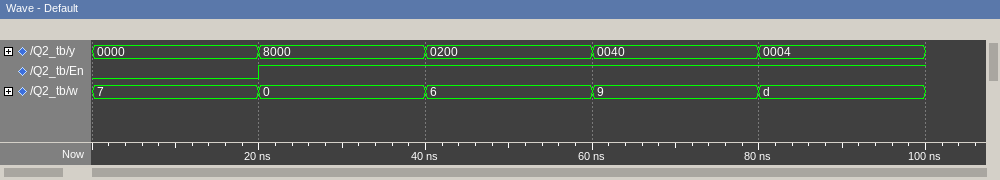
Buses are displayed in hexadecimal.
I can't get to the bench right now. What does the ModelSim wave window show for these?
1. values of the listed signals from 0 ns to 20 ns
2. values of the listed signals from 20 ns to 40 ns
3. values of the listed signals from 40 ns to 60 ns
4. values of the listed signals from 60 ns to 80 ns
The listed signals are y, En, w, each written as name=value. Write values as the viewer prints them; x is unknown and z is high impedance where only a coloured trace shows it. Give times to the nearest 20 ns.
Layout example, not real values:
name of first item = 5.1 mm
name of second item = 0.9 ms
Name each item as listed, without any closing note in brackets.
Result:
values of the listed signals from 0 ns to 20 ns = y=0000, En=0, w=7
values of the listed signals from 20 ns to 40 ns = y=8000, En=1, w=0
values of the listed signals from 40 ns to 60 ns = y=0200, En=1, w=6
values of the listed signals from 60 ns to 80 ns = y=0040, En=1, w=9
